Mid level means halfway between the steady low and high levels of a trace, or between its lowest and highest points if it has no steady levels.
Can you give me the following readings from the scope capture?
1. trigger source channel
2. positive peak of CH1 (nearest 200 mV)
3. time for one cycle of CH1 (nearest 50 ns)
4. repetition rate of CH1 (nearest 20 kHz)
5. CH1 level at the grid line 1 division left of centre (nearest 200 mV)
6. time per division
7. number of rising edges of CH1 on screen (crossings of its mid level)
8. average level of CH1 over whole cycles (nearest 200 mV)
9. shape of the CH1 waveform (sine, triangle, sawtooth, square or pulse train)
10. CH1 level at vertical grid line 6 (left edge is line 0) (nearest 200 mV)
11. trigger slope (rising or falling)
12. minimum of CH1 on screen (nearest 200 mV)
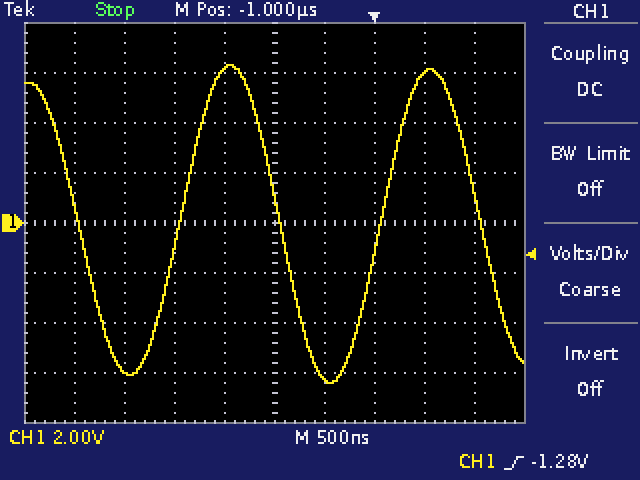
CH1
6.4 V
2.00 µs
500 kHz
6.2 V
500 ns
2
0.0 V
sine
-6.2 V
rising
-6.4 V
